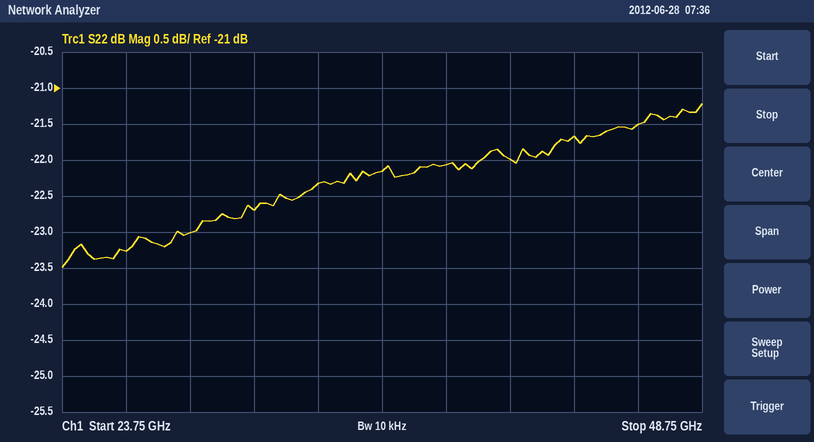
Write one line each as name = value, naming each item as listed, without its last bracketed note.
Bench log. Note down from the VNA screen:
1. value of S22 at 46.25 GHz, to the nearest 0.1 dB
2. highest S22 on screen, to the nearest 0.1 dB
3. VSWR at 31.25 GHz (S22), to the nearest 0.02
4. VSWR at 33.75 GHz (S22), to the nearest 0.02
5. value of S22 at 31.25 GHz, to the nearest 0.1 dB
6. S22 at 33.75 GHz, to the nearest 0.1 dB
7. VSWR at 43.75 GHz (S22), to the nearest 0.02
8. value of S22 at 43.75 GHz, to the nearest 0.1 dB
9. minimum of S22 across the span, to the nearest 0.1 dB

value of S22 at 46.25 GHz, to the nearest 0.1 dB = -21.5 dB
highest S22 on screen, to the nearest 0.1 dB = -21.2 dB
VSWR at 31.25 GHz (S22), to the nearest 0.02 = 1.16
VSWR at 33.75 GHz (S22), to the nearest 0.02 = 1.16
value of S22 at 31.25 GHz, to the nearest 0.1 dB = -22.7 dB
S22 at 33.75 GHz, to the nearest 0.1 dB = -22.3 dB
VSWR at 43.75 GHz (S22), to the nearest 0.02 = 1.18
value of S22 at 43.75 GHz, to the nearest 0.1 dB = -21.7 dB
minimum of S22 across the span, to the nearest 0.1 dB = -23.5 dB
